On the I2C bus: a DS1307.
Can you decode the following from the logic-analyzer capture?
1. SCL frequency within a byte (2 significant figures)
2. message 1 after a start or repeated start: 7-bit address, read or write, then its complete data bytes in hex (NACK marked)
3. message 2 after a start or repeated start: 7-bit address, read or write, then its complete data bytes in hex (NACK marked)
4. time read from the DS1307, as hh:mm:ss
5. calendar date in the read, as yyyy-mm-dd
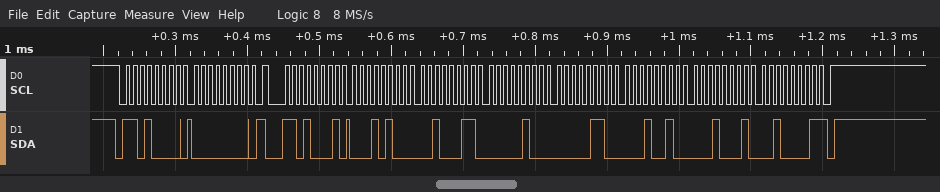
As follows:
100 kHz
0x68 write: 00
0x68 read: 14 23 04 06 12 11 21 NACK
04:23:14
2021-11-12
